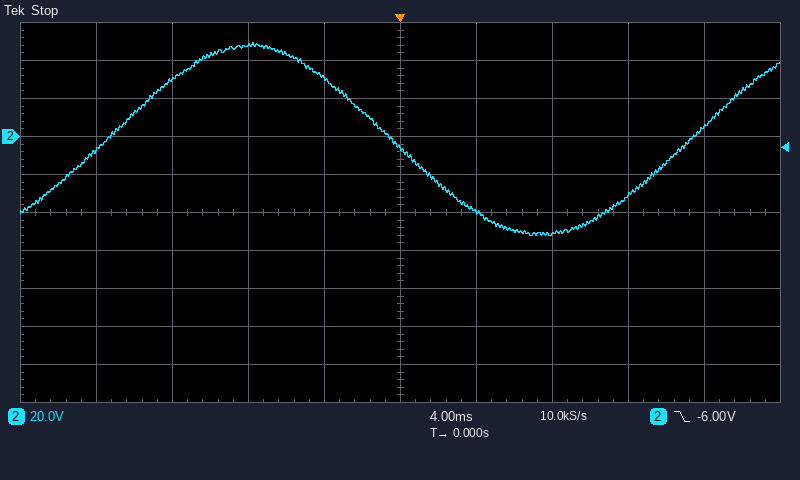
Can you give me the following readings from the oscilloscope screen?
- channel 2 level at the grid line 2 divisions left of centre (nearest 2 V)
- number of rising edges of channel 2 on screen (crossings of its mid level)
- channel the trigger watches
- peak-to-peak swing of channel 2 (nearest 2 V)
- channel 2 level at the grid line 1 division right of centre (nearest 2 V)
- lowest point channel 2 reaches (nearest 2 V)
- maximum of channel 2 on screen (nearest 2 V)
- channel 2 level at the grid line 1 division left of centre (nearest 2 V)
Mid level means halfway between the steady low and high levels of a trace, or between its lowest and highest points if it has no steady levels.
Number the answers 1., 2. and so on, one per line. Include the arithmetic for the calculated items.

1. 48 V
2. 2
3. channel 2
4. 50 V − (-52 V) = 102 V
5. -40 V
6. -52 V
7. 50 V
8. 30 V
